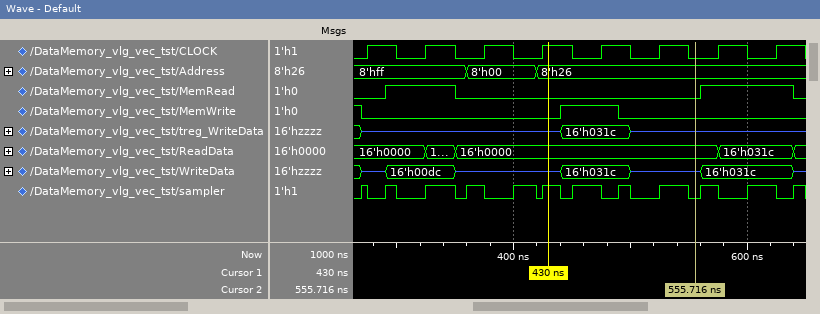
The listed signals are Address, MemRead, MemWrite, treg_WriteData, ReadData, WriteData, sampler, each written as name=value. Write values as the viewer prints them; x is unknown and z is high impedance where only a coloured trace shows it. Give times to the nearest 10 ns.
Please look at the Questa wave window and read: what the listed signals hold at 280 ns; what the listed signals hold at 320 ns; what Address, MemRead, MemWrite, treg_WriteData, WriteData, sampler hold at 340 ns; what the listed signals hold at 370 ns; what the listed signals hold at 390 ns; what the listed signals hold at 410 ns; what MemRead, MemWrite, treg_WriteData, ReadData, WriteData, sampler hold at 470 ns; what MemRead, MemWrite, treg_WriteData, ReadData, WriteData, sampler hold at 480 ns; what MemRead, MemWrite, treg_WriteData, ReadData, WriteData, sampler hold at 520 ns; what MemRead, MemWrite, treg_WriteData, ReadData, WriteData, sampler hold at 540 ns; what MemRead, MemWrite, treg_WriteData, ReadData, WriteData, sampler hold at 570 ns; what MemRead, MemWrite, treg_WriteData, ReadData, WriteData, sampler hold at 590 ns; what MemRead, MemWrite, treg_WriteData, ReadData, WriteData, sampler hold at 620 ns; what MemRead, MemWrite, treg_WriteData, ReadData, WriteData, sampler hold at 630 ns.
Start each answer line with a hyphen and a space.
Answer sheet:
- Address=8'hff, MemRead=0, MemWrite=0, treg_WriteData=z, ReadData=16'h0000, WriteData=z, sampler=0
- Address=8'hff, MemRead=1, MemWrite=0, treg_WriteData=z, ReadData=16'h0000, WriteData=16'h00dc, sampler=0
- Address=8'hff, MemRead=1, MemWrite=0, treg_WriteData=z, WriteData=16'h00dc, sampler=1
- Address=8'h00, MemRead=0, MemWrite=0, treg_WriteData=z, ReadData=16'h0000, WriteData=z, sampler=1
- Address=8'h00, MemRead=0, MemWrite=0, treg_WriteData=z, ReadData=16'h0000, WriteData=z, sampler=0
- Address=8'h00, MemRead=0, MemWrite=0, treg_WriteData=z, ReadData=16'h0000, WriteData=z, sampler=1
- MemRead=0, MemWrite=1, treg_WriteData=16'h031c, ReadData=16'h0000, WriteData=16'h031c, sampler=1
- MemRead=0, MemWrite=1, treg_WriteData=16'h031c, ReadData=16'h0000, WriteData=16'h031c, sampler=0
- MemRead=0, MemWrite=0, treg_WriteData=z, ReadData=16'h0000, WriteData=z, sampler=0
- MemRead=0, MemWrite=0, treg_WriteData=z, ReadData=16'h0000, WriteData=z, sampler=1
- MemRead=1, MemWrite=0, treg_WriteData=z, ReadData=16'h0000, WriteData=16'h031c, sampler=1
- MemRead=1, MemWrite=0, treg_WriteData=z, ReadData=16'h031c, WriteData=16'h031c, sampler=0
- MemRead=1, MemWrite=0, treg_WriteData=z, ReadData=16'h031c, WriteData=16'h031c, sampler=1
- MemRead=1, MemWrite=0, treg_WriteData=z, ReadData=16'h031c, WriteData=16'h031c, sampler=0
